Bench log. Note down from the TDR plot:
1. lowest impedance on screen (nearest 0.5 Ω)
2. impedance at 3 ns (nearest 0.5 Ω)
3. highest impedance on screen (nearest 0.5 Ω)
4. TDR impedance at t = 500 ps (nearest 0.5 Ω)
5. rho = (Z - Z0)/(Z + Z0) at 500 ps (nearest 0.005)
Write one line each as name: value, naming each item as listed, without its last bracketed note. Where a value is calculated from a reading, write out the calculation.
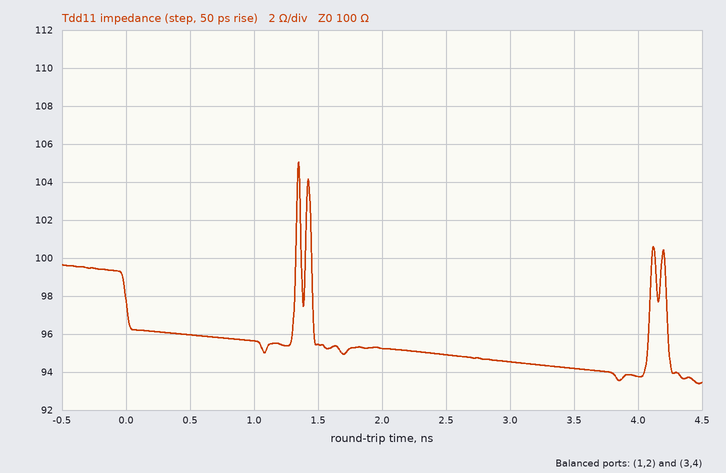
lowest impedance on screen: 93.5 Ω
impedance at 3 ns: 94.5 Ω
highest impedance on screen: 105.0 Ω
TDR impedance at t = 500 ps: 96.0 Ω
rho = (Z - Z0)/(Z + Z0) at 500 ps: (96 − 100)/(96 + 100) ≈ -0.020
